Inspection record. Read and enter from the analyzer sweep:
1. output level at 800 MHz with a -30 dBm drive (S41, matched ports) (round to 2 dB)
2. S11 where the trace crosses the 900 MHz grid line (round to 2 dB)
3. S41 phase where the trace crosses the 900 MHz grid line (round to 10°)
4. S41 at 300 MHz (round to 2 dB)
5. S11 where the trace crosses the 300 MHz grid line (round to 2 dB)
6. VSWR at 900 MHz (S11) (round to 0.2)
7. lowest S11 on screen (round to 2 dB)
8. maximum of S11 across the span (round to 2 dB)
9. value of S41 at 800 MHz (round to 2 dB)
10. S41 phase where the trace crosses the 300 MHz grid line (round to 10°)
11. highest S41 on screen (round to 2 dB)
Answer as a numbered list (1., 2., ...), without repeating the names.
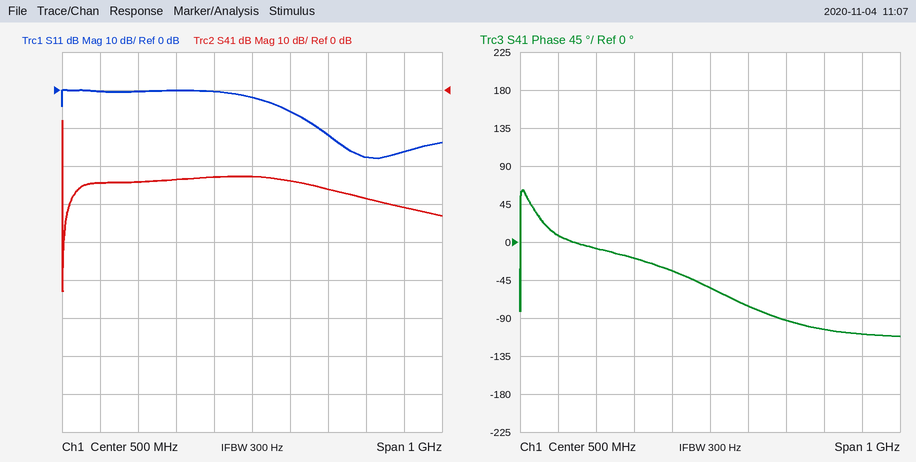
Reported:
1. -58 dBm
2. -16 dB
3. -110°
4. -24 dB
5. 0 dB
6. 1.4
7. -18 dB
8. 0 dB
9. -28 dB
10. -20°
11. -8 dB
